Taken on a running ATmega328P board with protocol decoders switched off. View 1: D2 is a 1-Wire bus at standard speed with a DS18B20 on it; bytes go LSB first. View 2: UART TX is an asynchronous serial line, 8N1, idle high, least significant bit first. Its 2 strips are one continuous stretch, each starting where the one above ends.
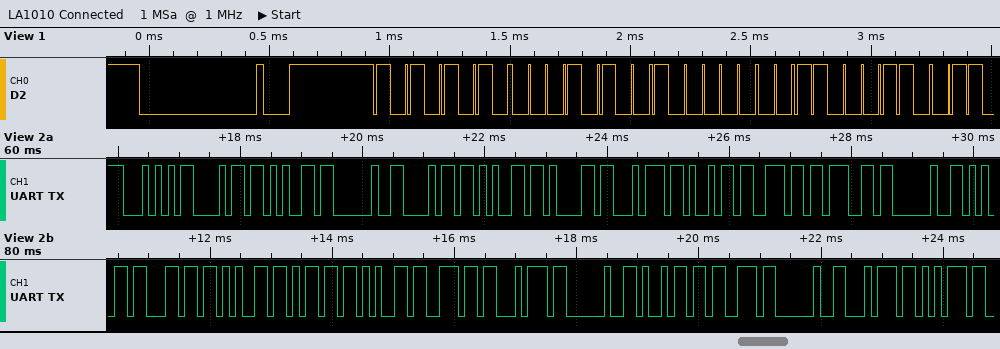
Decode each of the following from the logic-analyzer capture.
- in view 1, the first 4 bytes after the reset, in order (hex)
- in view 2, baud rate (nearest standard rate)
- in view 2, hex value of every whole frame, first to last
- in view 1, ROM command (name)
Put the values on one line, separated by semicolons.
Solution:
55 28 01 63; 9600 baud; 54 68 65 20 68 65 61 74 69 6E 67 20 65 6C 65 6D 65 6E 74 20 69 73 20 74 75; Match ROM
